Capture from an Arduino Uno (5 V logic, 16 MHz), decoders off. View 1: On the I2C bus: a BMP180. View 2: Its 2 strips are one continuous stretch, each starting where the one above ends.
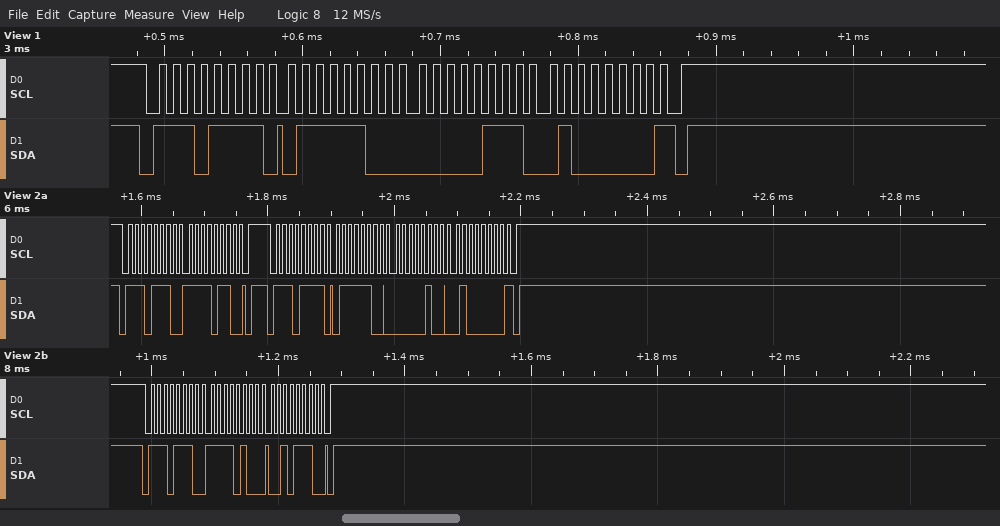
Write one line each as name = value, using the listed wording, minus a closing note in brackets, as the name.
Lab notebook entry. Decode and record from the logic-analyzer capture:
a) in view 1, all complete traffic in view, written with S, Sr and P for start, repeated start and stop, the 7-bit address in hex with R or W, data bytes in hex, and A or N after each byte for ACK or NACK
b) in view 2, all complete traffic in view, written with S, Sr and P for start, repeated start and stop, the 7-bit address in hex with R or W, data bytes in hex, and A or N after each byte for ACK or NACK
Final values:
in view 1, all complete traffic in view, written with S, Sr and P for start, repeated start and stop, the 7-bit address in hex with R or W, data bytes in hex, and A or N after each byte for ACK or NACK = S 77R A 7C A 07 A 40 N P
in view 2, all complete traffic in view, written with S, Sr and P for start, repeated start and stop, the 7-bit address in hex with R or W, data bytes in hex, and A or N after each byte for ACK or NACK = S 77W A F6 A P S 77R A 7C A 04 A 40 N P S 77W A F4 A 2E A P
